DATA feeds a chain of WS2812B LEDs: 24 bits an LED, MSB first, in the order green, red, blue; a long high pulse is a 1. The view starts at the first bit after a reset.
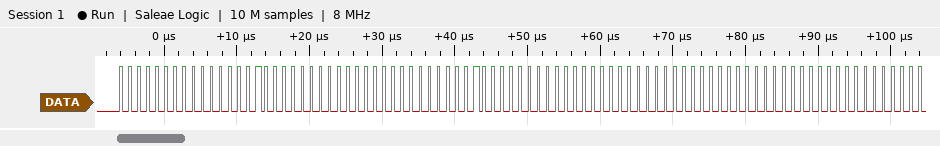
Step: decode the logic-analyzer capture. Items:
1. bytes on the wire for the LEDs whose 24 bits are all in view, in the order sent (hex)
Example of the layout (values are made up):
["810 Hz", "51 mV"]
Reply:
["00 01 00 00 01 00 00 00 00"]
